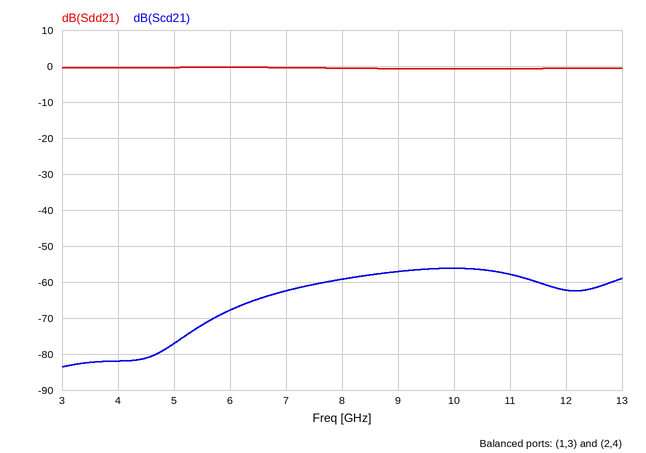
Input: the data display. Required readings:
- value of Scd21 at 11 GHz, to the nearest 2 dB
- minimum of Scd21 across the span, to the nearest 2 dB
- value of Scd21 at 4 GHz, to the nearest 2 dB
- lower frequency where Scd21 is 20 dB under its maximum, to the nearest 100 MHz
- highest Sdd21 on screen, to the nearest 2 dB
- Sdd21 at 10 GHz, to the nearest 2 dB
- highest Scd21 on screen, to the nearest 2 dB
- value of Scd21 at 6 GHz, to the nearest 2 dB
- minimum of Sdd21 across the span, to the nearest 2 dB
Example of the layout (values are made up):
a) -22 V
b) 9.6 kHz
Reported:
a) -58 dB
b) -84 dB
c) -82 dB
d) 5.1 GHz
e) 0 dB
f) 0 dB
g) -56 dB
h) -68 dB
i) 0 dB
